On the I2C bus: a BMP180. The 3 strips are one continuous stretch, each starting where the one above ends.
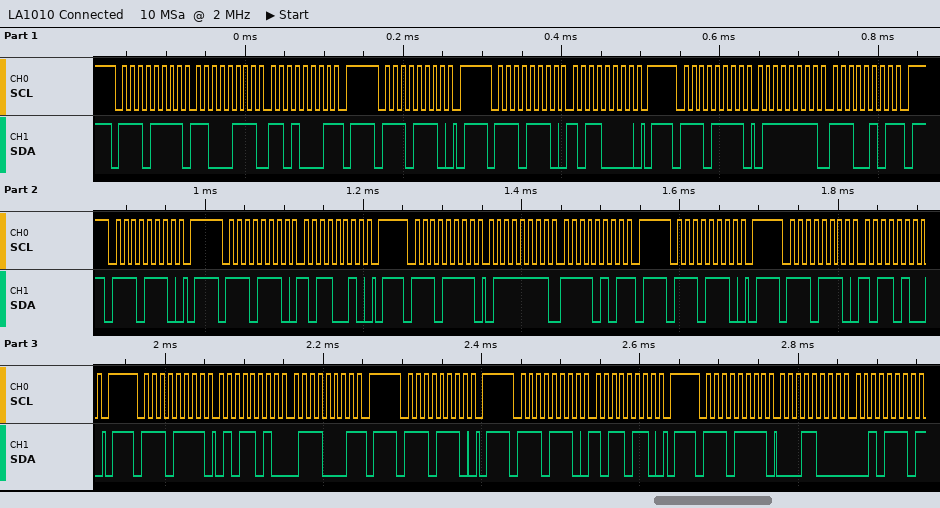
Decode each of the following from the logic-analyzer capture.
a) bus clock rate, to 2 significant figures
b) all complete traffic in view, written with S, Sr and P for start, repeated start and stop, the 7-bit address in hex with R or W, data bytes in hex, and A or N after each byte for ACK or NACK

100 kHz
S 77R A C7 A D1 N P S 77W A P S 77W A B0 A P S 77R A 7F A E5 N P S 77W A P S 77W A B2 A P S 77R A 7F A F5 N P S 77W A P S 77W A B4 A P S 77R A 5A A 71 N P S 77W A P S 77W A B6 A P S 77R A 18 A 2E N
